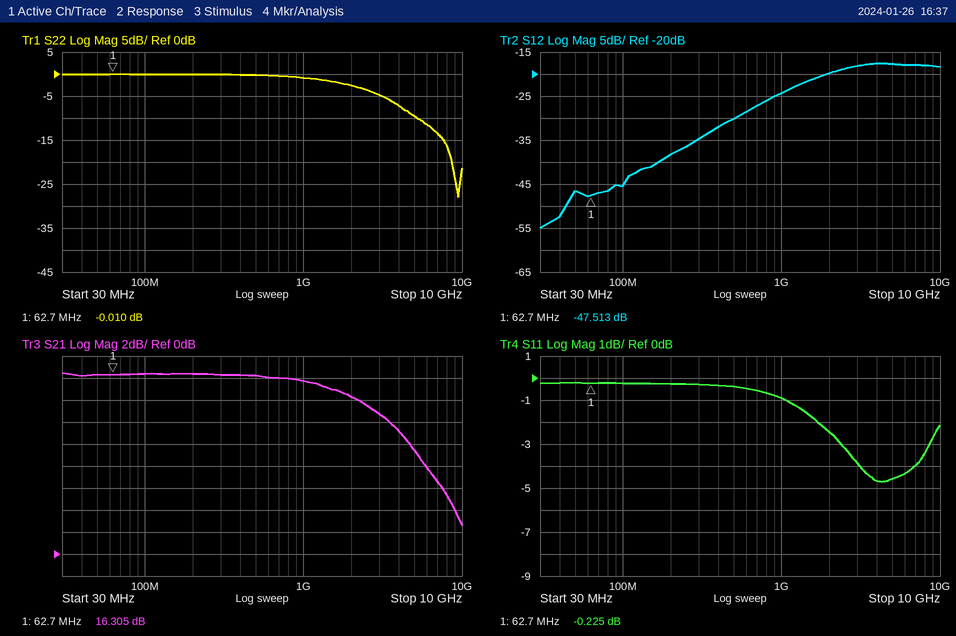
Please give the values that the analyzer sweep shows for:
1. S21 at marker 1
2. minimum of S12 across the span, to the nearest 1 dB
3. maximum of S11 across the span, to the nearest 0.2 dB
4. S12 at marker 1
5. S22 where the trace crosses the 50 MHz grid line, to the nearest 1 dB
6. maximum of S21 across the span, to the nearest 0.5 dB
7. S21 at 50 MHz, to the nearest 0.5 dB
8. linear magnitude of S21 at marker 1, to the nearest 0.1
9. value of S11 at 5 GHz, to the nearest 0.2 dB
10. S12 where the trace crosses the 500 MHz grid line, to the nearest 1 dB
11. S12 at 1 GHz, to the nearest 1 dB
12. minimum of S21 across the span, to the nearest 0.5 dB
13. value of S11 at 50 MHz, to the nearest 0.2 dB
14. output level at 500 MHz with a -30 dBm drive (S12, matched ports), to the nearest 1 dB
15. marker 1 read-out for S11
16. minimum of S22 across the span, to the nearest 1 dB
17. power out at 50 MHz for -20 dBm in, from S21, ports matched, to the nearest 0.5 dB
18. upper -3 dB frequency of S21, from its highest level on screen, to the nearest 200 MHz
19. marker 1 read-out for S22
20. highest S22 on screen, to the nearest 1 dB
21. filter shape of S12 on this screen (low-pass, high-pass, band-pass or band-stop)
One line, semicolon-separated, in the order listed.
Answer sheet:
16.305 dB; -55 dB; -0.2 dB; -47.513 dB; 0 dB; 16.5 dB; 16.5 dB; 6.5; -4.6 dB; -30 dB; -24 dB; 2.5 dB; -0.2 dB; -60 dBm; -0.225 dB; -28 dB; -3.5 dBm; 2.6 GHz; -0.010 dB; 0 dB; high-pass
